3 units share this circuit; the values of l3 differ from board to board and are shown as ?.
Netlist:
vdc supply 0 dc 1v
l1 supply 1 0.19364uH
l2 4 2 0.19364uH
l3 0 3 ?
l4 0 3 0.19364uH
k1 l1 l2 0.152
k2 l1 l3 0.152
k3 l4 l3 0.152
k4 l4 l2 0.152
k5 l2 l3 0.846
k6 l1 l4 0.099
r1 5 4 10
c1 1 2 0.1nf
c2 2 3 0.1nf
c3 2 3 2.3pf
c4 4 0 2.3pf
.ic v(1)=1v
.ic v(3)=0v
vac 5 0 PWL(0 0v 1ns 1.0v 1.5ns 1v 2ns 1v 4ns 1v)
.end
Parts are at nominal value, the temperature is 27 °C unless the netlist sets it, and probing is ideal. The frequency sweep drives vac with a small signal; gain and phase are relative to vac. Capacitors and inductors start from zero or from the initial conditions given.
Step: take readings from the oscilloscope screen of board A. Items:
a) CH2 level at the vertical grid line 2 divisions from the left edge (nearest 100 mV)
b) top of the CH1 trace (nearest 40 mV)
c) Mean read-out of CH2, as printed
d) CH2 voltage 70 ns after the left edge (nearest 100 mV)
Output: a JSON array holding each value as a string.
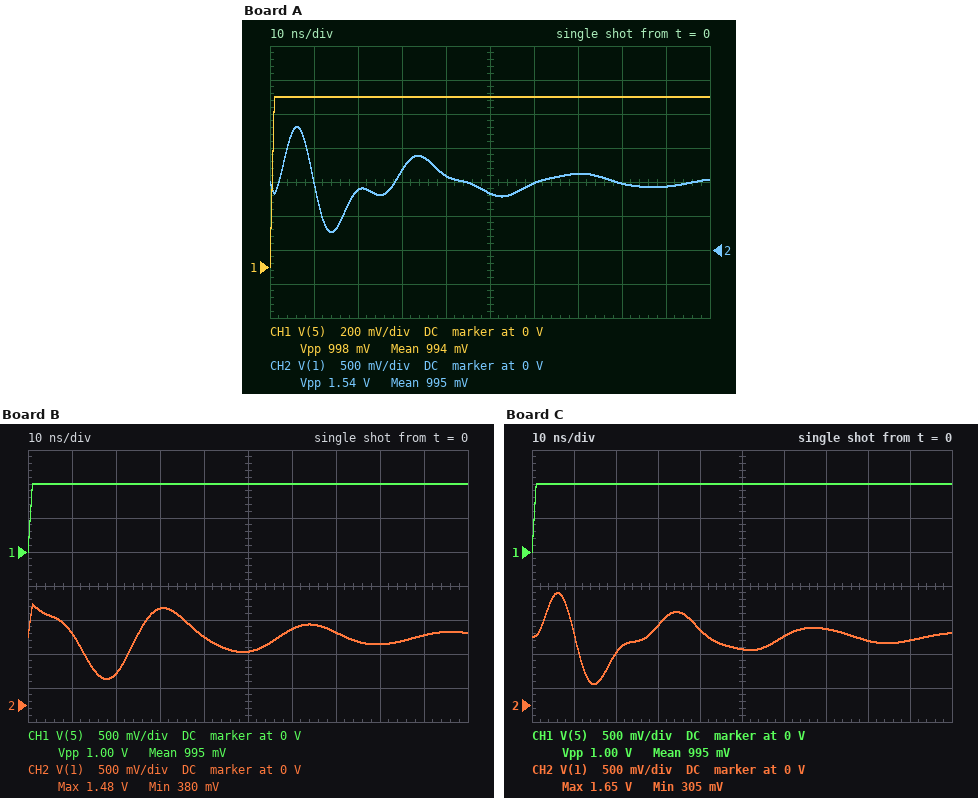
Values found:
["900 mV", "1.00 V", "995 mV", "1.1 V"]
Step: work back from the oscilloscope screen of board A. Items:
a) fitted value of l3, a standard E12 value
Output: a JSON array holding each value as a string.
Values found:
["100 nH"]
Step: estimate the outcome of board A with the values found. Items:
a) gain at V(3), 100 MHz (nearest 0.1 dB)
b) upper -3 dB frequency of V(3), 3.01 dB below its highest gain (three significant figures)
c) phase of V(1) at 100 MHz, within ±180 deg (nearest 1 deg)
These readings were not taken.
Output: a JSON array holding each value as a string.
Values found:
["-15.8 dB", "34.5 MHz", "-151 deg"]
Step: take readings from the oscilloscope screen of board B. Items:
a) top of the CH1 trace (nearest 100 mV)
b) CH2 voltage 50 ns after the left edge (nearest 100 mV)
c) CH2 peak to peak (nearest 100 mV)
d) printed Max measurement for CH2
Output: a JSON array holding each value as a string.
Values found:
["1.0 V", "800 mV", "1.1 V", "1.48 V"]
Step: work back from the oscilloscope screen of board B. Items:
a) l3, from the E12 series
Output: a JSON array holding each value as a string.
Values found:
["390 nH"]
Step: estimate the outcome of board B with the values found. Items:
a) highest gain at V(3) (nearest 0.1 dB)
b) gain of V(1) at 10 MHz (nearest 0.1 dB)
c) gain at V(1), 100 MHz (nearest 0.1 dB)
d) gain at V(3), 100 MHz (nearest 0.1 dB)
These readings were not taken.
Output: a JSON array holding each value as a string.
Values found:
["9.0 dB", "-22.1 dB", "-6.6 dB", "-1.5 dB"]
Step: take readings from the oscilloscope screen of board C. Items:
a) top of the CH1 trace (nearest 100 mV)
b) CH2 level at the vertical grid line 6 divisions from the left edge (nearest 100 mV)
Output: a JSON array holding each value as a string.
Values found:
["1.0 V", "1.0 V"]
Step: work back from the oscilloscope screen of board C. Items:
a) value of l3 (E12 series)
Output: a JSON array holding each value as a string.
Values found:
["150 nH"]
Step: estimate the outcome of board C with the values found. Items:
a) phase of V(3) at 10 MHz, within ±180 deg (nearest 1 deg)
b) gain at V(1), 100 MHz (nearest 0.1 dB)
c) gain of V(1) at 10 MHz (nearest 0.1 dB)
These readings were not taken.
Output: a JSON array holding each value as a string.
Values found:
["-8 deg", "-3.9 dB", "-22.7 dB"]
